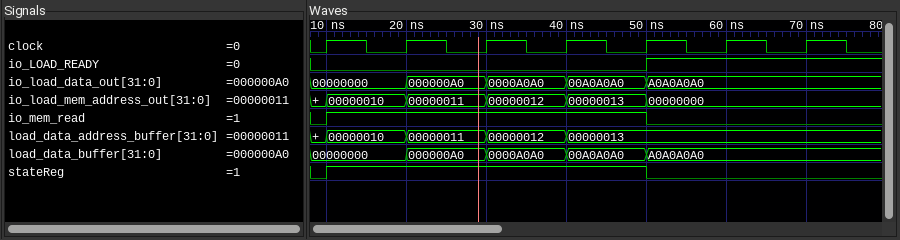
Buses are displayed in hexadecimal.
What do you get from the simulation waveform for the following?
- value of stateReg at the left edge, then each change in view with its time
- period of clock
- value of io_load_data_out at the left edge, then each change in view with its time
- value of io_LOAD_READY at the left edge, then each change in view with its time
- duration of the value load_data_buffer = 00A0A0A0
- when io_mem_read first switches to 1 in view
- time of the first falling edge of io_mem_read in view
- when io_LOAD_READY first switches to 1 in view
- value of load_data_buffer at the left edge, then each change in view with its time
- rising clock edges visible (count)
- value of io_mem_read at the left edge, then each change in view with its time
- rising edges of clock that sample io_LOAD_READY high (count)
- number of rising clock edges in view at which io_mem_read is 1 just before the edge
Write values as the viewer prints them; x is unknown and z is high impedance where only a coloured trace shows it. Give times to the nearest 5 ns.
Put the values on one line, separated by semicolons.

0, 1 at 10 ns, 0 at 50 ns; 10 ns; 00000000, 000000A0 at 20 ns, 0000A0A0 at 30 ns, 00A0A0A0 at 40 ns, A0A0A0A0 at 50 ns; 0, 1 at 50 ns; 10 ns; 10 ns; 50 ns; 50 ns; 00000000, 000000A0 at 20 ns, 0000A0A0 at 30 ns, 00A0A0A0 at 40 ns, A0A0A0A0 at 50 ns; 7; 0, 1 at 10 ns, 0 at 50 ns; 2; 4
